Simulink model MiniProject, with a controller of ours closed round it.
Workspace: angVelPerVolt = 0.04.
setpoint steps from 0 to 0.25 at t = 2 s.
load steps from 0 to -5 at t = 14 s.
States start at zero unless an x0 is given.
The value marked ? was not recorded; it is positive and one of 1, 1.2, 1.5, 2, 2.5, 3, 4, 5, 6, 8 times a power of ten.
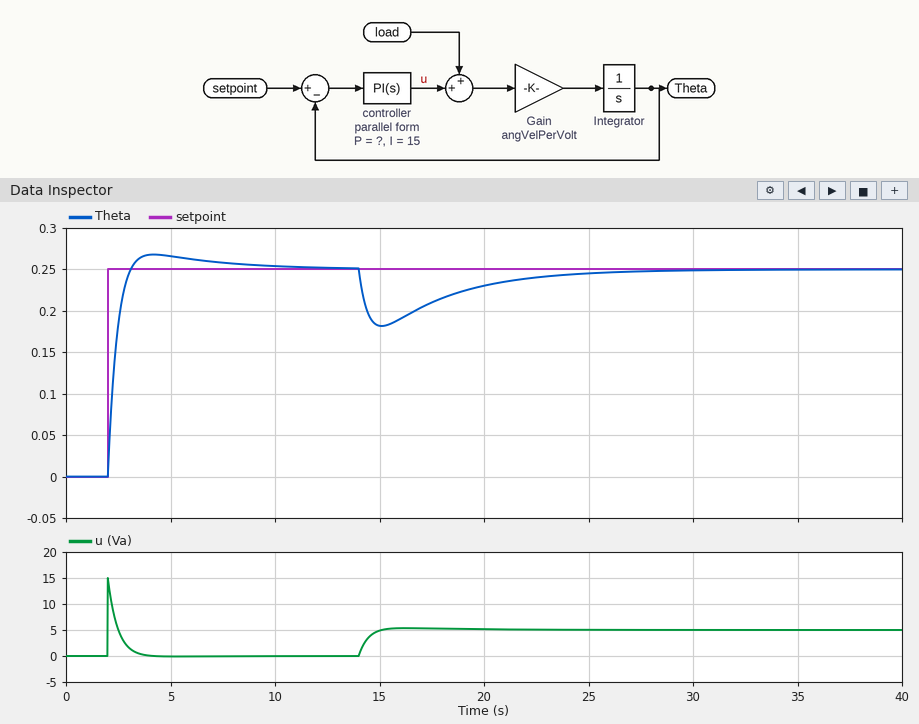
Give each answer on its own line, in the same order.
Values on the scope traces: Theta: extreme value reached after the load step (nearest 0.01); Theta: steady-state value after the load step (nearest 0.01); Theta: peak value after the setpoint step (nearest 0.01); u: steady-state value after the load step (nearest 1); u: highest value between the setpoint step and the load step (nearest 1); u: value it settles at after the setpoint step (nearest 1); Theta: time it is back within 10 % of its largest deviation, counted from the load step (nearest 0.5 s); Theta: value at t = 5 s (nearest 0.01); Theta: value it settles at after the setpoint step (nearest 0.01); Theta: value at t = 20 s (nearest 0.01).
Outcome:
0.18
0.25
0.27
5
15
0
9.5 s
0.27
0.25
0.23
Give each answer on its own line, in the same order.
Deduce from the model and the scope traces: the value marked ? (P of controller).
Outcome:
60
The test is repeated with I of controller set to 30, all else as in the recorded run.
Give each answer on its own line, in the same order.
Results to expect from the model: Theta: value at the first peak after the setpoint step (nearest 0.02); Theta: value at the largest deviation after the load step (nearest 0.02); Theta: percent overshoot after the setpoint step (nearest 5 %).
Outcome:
0.28
0.18
10 %
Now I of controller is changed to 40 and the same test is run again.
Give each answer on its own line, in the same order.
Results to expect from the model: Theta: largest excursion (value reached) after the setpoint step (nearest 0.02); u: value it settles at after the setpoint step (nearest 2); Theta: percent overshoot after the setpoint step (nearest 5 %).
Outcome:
0.28
0
15 %
